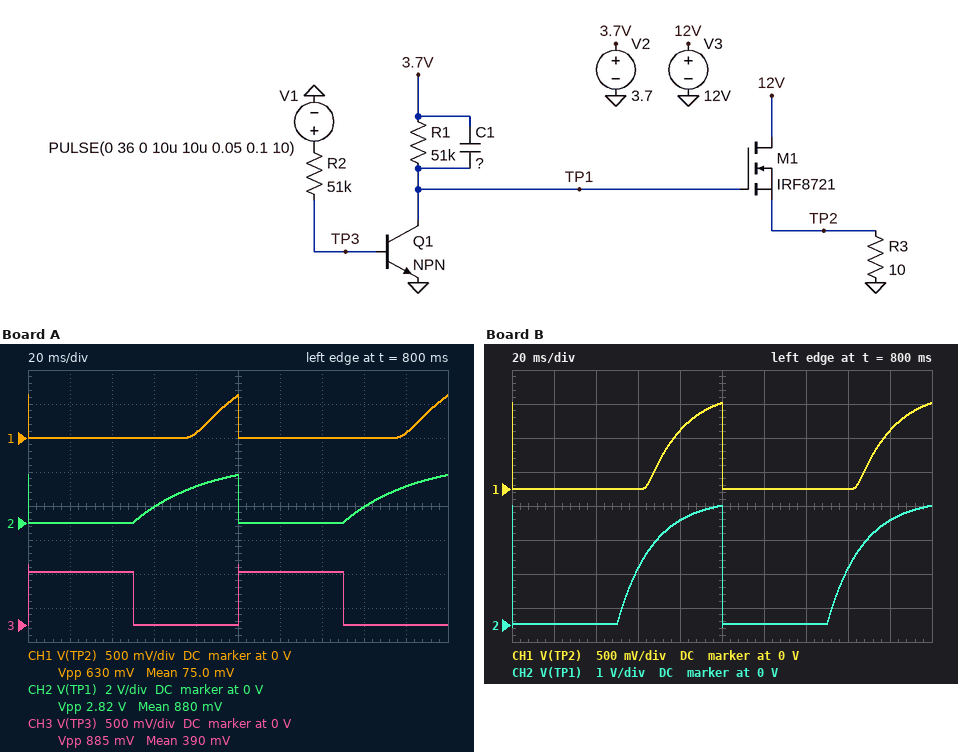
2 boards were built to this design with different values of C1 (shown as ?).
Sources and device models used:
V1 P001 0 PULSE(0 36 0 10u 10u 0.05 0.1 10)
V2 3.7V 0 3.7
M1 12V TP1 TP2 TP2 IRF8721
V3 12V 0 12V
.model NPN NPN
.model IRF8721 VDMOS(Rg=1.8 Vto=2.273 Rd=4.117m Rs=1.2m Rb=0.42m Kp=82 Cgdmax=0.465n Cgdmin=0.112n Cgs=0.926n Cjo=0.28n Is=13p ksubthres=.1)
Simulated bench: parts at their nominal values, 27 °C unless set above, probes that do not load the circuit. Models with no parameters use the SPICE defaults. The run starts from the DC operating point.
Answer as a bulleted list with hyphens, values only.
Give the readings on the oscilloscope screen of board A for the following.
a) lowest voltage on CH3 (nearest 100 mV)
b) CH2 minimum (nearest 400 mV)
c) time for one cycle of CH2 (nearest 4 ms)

- 0 V
- 0 V
- 100 ms
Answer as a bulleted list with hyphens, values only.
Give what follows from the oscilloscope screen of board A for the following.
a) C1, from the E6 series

- 680 nF
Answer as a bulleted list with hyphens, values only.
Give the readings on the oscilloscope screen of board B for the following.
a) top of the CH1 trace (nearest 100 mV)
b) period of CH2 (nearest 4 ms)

- 1.3 V
- 100 ms
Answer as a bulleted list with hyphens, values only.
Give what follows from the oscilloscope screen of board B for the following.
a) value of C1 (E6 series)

- 330 nF
